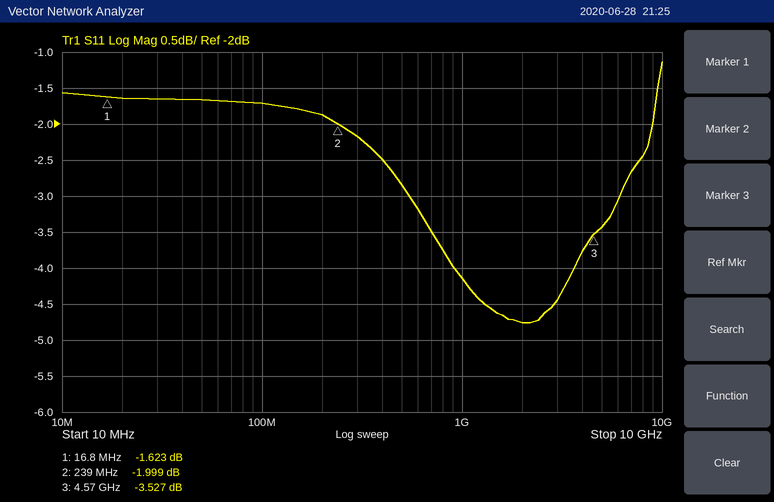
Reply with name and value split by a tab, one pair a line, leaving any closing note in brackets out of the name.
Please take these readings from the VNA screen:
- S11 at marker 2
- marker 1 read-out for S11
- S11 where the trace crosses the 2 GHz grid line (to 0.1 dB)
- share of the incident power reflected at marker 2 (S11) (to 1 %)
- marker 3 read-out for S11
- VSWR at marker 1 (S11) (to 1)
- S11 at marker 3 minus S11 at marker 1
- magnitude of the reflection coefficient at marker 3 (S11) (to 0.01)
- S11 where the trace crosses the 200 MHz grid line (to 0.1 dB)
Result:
S11 at marker 2	-1.999 dB
marker 1 read-out for S11	-1.623 dB
S11 where the trace crosses the 2 GHz grid line	-4.8 dB
share of the incident power reflected at marker 2 (S11)	63 %
marker 3 read-out for S11	-3.527 dB
VSWR at marker 1 (S11)	11
S11 at marker 3 minus S11 at marker 1	-1.904 dB
magnitude of the reflection coefficient at marker 3 (S11)	0.67
S11 where the trace crosses the 200 MHz grid line	-1.9 dB
